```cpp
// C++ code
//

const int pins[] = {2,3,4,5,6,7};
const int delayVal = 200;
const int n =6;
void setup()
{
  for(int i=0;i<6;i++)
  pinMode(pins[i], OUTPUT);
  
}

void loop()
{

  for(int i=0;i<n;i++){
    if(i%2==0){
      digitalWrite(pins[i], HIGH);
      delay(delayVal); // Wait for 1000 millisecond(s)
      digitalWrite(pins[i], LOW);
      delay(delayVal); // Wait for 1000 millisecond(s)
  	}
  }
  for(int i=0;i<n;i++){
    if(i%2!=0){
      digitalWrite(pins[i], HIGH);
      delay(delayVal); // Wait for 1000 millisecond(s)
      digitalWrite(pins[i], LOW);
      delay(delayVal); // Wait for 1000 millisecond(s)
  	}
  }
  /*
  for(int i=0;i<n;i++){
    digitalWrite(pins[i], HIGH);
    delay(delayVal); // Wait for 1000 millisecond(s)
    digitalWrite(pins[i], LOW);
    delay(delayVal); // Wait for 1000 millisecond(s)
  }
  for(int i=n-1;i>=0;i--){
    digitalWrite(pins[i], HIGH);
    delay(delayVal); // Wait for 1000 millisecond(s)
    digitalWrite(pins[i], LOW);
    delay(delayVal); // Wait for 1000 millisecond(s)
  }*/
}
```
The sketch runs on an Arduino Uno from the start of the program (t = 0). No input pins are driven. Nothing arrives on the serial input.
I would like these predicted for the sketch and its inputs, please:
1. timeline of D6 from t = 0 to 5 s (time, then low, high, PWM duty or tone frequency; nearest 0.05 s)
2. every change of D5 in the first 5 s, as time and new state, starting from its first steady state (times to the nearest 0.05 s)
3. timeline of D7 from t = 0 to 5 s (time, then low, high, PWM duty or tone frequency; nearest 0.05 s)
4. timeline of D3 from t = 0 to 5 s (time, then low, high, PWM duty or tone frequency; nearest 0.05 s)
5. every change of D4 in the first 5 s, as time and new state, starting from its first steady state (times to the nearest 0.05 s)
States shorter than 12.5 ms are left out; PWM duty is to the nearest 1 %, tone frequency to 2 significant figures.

0 s low; 0.8 s high; 1 s low; 3.2 s high; 3.4 s low
0 s low; 1.6 s high; 1.8 s low; 4 s high; 4.2 s low
0 s low; 2 s high; 2.2 s low; 4.4 s high; 4.6 s low
0 s low; 1.2 s high; 1.4 s low; 3.6 s high; 3.8 s low
0 s low; 0.4 s high; 0.6 s low; 2.8 s high; 3 s low
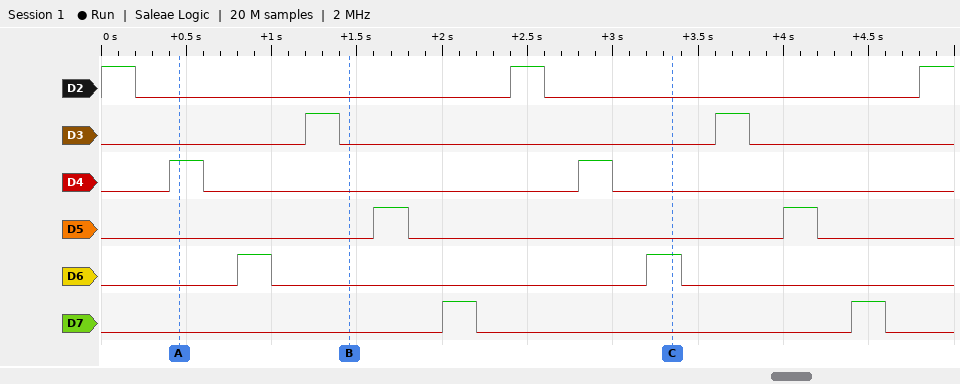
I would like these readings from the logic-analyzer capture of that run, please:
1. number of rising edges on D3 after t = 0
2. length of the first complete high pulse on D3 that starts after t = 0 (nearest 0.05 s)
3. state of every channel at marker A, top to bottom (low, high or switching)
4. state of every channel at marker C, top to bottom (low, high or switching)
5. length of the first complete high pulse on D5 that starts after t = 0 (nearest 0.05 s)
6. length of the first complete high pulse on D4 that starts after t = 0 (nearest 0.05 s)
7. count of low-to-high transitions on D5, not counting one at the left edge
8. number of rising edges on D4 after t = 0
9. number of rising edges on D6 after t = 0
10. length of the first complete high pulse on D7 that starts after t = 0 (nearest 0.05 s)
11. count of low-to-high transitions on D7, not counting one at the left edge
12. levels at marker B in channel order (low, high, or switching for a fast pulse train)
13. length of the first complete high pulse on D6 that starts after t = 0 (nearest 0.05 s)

2
0.20 s
D2 low, D3 low, D4 high, D5 low, D6 low, D7 low
D2 low, D3 low, D4 low, D5 low, D6 high, D7 low
0.20 s
0.20 s
2
2
2
0.20 s
2
D2 low, D3 low, D4 low, D5 low, D6 low, D7 low
0.20 s
